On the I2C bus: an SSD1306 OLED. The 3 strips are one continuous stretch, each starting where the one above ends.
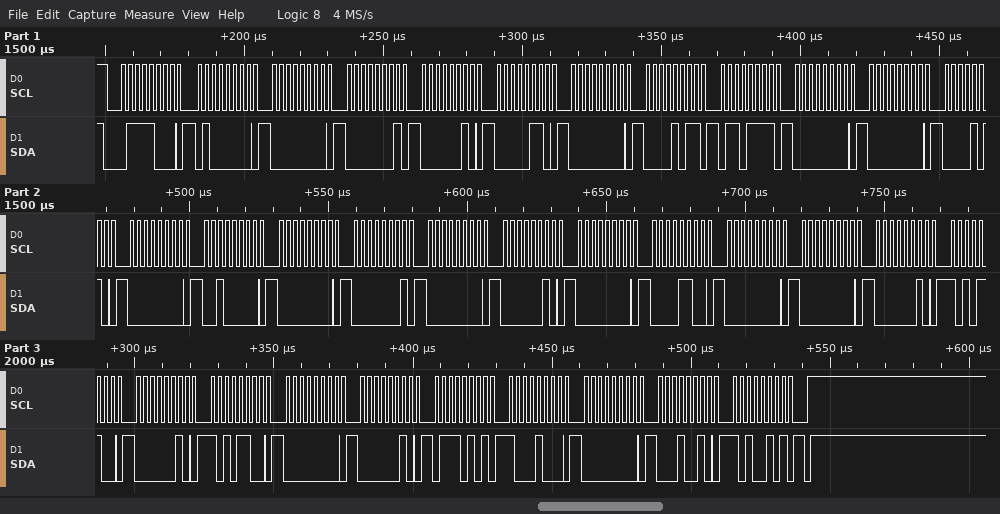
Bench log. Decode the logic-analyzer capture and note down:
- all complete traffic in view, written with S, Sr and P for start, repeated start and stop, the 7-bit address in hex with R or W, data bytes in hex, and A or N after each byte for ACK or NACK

S 3CW A 40 A 00 A 01 A 02 A 06 A 00 A 0B A 6F A 00 A 00 A 0A A 00 A 20 A 00 A 01 A 00 A 02 A 00 A 0C A 00 A 00 A 02 A AC A 02 A AC A 00 A 02 A 75 A 88 A 00 A 12 A A5 A P
